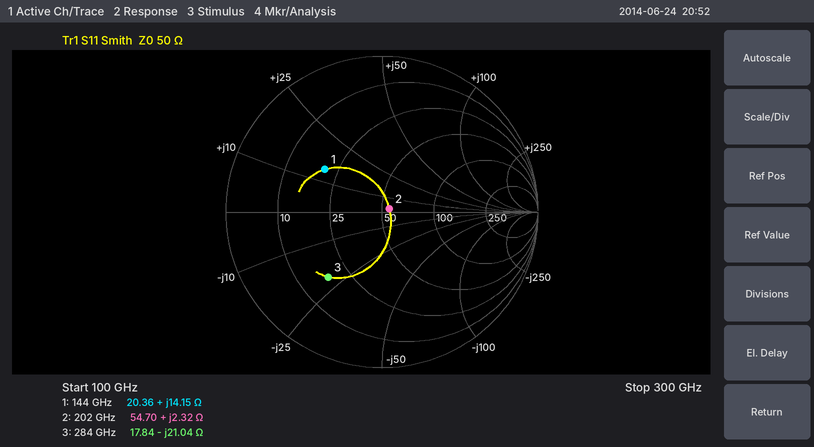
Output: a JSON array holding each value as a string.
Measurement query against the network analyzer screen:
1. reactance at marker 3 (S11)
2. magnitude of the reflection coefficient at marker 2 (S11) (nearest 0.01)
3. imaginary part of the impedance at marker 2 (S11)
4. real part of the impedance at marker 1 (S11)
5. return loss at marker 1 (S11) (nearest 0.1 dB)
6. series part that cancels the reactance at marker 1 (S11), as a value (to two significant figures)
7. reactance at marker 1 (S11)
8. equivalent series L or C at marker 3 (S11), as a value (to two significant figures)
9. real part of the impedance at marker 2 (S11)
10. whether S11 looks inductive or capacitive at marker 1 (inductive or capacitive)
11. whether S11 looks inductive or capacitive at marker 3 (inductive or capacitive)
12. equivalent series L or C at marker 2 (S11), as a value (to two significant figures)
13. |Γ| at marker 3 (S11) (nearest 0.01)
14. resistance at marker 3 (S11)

["-21.04 Ω", "0.05", "+2.32 Ω", "20.36 Ω", "6.8 dB", "78 fF", "+14.15 Ω", "27 fF", "54.70 Ω", "inductive", "capacitive", "1.8 pH", "0.54", "17.84 Ω"]
